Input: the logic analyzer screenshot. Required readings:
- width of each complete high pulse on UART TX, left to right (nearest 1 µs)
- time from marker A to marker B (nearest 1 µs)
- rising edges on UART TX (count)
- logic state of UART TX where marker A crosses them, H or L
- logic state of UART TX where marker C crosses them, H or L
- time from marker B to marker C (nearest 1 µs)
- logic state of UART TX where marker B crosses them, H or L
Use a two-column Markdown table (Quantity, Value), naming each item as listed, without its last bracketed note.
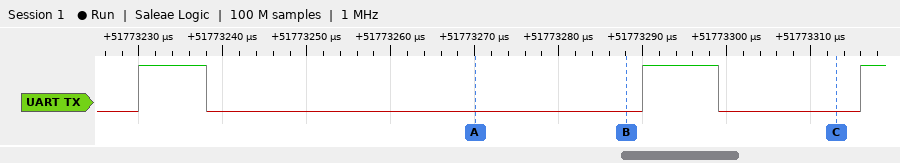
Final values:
| Quantity | Value |
|---|---|
| width of each complete high pulse on UART TX, left to right | 8 µs, 9 µs |
| time from marker A to marker B | 18 µs |
| rising edges on UART TX | 3 |
| logic state of UART TX where marker A crosses them, H or L | UART TX=L |
| logic state of UART TX where marker C crosses them, H or L | UART TX=L |
| time from marker B to marker C | 25 µs |
| logic state of UART TX where marker B crosses them, H or L | UART TX=L |
